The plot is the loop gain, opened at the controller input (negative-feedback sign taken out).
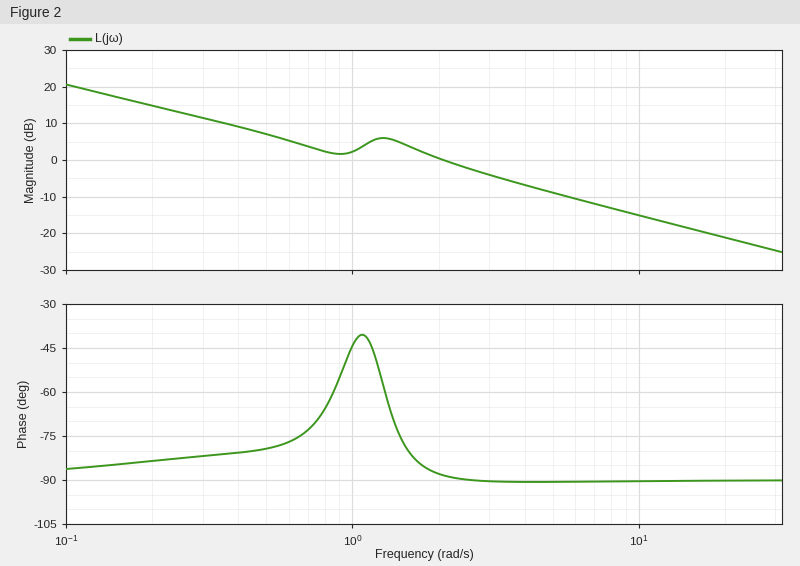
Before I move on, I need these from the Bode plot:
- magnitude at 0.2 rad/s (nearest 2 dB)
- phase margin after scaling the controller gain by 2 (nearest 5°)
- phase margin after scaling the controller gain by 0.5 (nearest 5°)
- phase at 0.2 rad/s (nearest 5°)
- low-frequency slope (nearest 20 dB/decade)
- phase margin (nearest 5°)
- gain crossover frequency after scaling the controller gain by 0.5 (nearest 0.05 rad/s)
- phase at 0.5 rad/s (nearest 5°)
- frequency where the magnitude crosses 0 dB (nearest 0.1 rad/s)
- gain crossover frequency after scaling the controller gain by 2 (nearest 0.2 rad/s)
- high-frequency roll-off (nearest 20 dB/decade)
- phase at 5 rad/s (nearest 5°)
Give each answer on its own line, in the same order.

14 dB
90°
100°
-85°
-20 dB/decade
90°
0.55 rad/s
-80°
2.1 rad/s
3.6 rad/s
-20 dB/decade
-90°
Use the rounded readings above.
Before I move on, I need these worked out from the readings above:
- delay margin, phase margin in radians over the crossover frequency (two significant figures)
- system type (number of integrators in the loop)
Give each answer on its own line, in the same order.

0.75 s
1
